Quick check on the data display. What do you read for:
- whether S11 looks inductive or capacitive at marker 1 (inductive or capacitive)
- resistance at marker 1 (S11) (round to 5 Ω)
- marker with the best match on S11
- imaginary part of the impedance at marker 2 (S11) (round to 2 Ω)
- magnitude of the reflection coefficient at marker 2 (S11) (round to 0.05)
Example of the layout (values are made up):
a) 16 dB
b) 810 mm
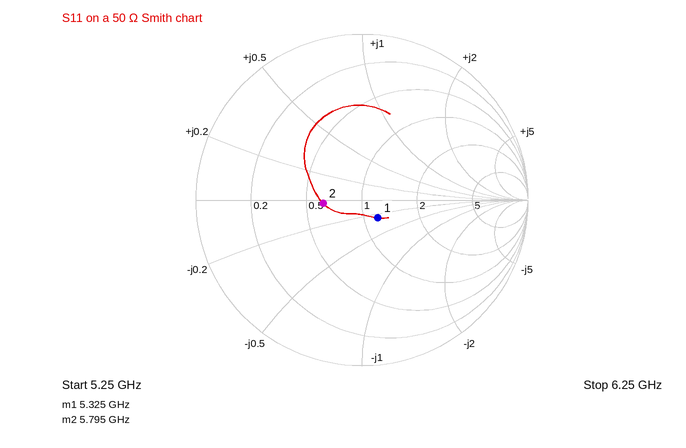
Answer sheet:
a) capacitive
b) 60 Ω
c) marker 1
d) -2 Ω
e) 0.25
